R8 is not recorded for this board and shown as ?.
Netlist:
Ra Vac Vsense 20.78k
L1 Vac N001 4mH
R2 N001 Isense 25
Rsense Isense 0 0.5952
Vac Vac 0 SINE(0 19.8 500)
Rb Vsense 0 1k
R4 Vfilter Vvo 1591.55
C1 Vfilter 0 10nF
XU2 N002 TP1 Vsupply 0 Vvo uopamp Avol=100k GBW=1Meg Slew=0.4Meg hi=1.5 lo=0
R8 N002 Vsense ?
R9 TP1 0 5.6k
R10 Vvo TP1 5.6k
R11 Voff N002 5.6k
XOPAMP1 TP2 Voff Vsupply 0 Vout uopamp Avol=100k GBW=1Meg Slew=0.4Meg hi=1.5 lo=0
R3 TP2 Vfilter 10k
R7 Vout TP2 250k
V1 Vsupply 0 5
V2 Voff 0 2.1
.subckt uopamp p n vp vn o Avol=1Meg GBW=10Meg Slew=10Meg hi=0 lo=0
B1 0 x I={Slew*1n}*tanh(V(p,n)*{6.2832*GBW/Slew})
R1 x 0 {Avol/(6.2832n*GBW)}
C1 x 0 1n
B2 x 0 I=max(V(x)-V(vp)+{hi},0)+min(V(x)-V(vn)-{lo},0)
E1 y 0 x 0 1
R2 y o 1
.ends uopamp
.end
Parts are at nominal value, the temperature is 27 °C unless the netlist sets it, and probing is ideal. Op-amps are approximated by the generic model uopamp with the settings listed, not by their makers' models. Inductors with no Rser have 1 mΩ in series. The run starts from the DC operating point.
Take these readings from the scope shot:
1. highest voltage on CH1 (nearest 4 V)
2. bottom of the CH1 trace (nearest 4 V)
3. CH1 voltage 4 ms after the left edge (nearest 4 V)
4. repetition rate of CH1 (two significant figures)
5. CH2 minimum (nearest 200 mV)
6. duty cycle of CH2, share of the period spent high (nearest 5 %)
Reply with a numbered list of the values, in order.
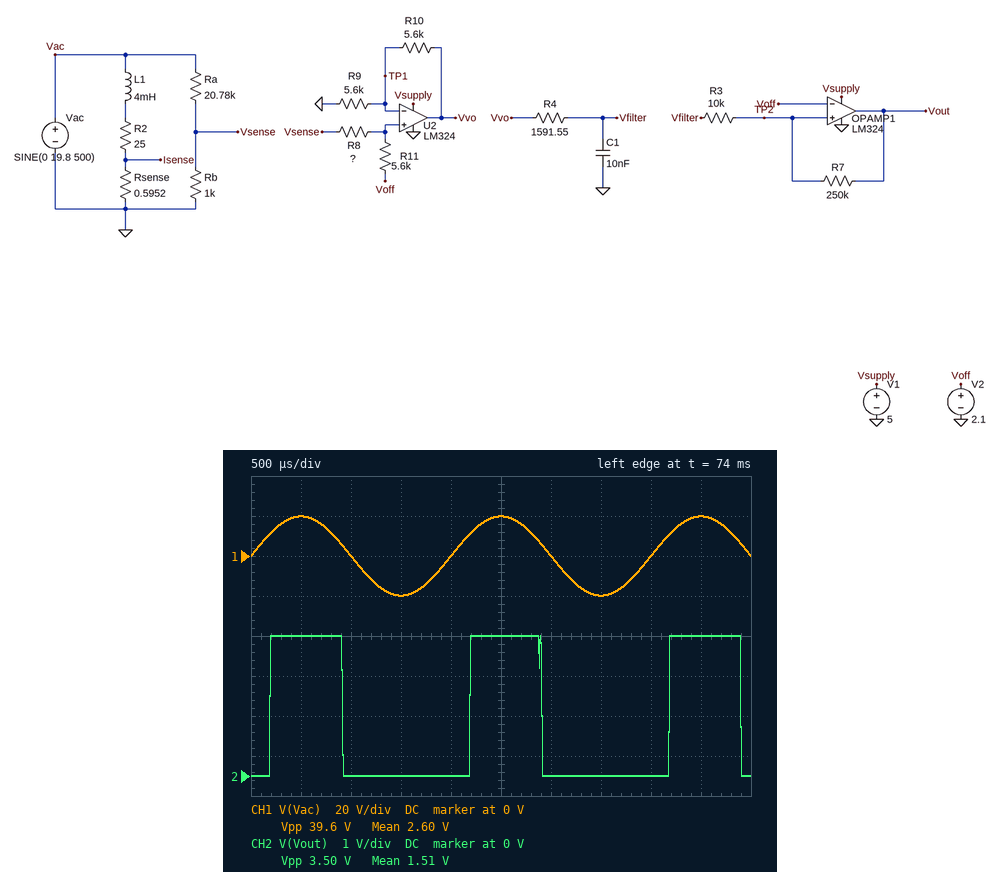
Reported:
1. 20 V
2. -20 V
3. 0 V
4. 500 Hz
5. 0 V
6. 35 %
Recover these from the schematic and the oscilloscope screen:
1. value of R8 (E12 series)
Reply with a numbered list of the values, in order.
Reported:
1. 2.7 kΩ
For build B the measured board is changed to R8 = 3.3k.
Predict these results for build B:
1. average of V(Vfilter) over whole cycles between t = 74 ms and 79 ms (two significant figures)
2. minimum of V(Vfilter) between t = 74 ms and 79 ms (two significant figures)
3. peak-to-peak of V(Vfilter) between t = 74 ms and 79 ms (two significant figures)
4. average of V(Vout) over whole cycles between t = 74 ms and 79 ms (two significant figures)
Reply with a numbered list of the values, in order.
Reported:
1. 1.8 V
2. 780 mV
3. 2.1 V
4. 1.4 V
